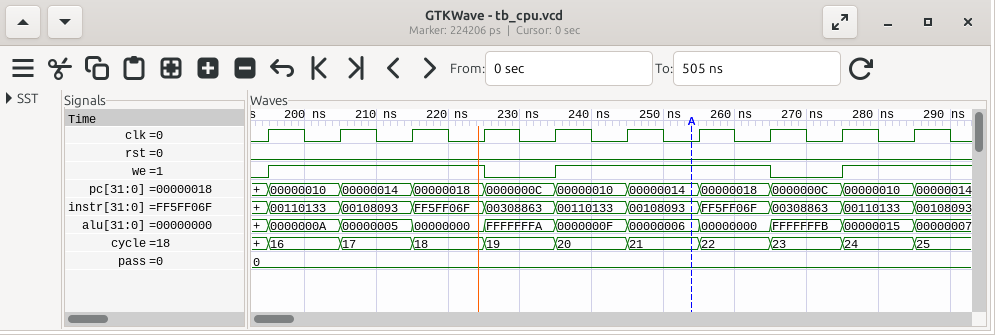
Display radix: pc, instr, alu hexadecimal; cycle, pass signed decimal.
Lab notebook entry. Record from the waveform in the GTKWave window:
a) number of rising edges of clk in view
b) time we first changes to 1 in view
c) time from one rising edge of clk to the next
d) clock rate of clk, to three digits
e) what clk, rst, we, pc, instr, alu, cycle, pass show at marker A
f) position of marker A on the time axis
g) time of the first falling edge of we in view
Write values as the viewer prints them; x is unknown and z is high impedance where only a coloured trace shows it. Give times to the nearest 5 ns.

10
195 ns
10 ns
100 MHz
clk=0, rst=0, we=1, pc=00000014, instr=00108093, alu=00000006, cycle=21, pass=0
255 ns
225 ns
